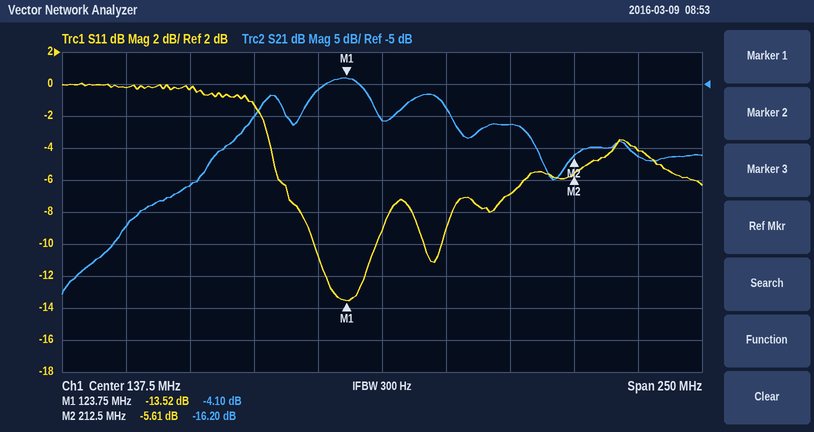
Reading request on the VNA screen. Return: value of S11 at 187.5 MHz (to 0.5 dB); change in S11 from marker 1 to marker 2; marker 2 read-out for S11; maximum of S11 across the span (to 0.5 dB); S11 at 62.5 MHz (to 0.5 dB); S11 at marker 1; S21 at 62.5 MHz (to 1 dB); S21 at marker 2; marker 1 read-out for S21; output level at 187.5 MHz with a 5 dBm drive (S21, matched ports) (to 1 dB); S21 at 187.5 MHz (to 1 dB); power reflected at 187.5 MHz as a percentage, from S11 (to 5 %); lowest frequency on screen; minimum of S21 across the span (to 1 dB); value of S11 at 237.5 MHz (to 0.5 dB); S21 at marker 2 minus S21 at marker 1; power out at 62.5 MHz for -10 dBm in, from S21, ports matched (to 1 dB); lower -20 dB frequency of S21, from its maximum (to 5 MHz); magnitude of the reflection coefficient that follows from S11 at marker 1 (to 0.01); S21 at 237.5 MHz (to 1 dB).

-7.0 dB
7.91 dB
-5.61 dB
0.0 dB
-0.5 dB
-13.52 dB
-21 dB
-16.20 dB
-4.10 dB
-6 dBm
-11 dB
20 %
12.5 MHz
-38 dB
-4.0 dB
-12.10 dB
-31 dBm
45 MHz
0.21
-16 dB
